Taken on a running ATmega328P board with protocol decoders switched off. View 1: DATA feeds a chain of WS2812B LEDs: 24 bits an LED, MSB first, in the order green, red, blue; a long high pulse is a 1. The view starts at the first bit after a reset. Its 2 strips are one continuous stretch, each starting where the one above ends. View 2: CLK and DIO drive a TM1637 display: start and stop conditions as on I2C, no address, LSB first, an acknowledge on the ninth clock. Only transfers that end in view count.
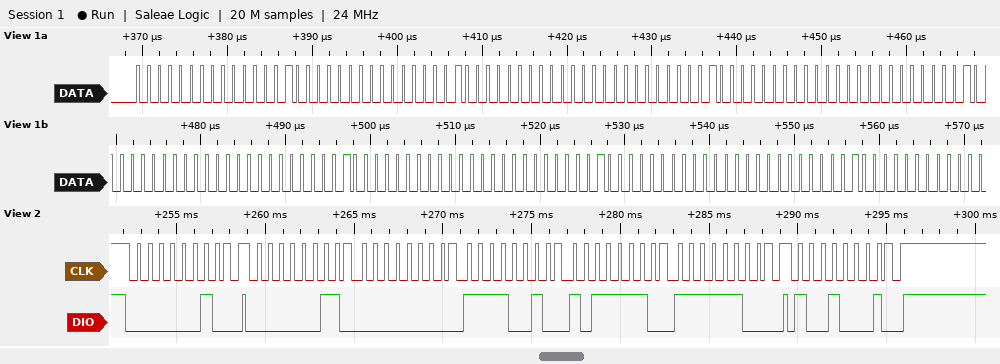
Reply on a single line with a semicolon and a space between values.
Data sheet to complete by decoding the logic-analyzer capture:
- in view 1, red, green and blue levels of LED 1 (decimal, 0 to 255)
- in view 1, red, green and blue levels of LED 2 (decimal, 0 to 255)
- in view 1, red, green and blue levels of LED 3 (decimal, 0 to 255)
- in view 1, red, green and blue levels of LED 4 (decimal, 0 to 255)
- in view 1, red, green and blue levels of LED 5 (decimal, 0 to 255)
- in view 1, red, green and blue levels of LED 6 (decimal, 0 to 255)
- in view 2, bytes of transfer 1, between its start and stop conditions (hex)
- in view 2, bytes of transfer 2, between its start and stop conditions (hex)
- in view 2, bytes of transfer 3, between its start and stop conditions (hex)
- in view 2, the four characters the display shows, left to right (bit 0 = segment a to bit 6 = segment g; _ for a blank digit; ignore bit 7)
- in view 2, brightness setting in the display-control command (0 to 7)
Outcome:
2, 0, 0; 0, 2, 0; 0, 2, 0; 0, 2, 0; 0, 2, 0; 0, 2, 0; 40; C0 00 4F 7D 3F; 89; _360; 1
